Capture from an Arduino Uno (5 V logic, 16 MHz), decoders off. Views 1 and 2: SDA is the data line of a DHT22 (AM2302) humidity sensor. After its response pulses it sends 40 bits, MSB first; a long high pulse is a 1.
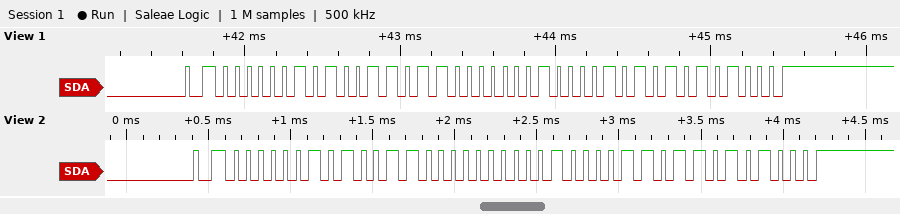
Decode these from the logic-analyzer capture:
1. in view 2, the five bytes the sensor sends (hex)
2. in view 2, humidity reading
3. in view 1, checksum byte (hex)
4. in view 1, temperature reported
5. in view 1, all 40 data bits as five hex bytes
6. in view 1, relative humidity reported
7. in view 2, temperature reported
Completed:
02 98 01 0D A8
66.4 %
0xA8
26.6 °C
02 9B 01 0A A8
66.7 %
26.9 °C
